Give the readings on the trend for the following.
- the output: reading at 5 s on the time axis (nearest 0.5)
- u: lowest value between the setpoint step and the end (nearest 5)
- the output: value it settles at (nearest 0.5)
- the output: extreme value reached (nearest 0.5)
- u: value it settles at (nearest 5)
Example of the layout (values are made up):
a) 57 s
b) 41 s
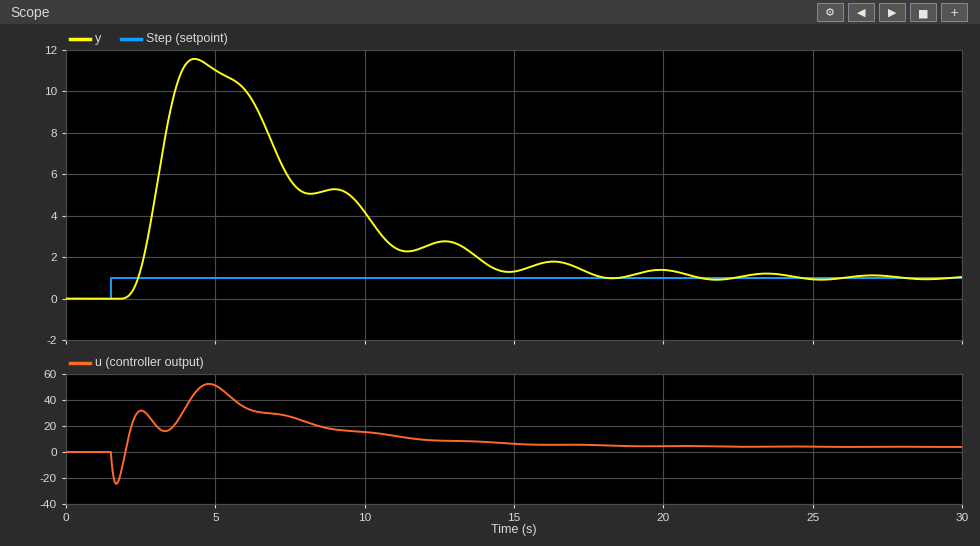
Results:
a) 11.0
b) -25
c) 1.0
d) 11.5
e) 5
